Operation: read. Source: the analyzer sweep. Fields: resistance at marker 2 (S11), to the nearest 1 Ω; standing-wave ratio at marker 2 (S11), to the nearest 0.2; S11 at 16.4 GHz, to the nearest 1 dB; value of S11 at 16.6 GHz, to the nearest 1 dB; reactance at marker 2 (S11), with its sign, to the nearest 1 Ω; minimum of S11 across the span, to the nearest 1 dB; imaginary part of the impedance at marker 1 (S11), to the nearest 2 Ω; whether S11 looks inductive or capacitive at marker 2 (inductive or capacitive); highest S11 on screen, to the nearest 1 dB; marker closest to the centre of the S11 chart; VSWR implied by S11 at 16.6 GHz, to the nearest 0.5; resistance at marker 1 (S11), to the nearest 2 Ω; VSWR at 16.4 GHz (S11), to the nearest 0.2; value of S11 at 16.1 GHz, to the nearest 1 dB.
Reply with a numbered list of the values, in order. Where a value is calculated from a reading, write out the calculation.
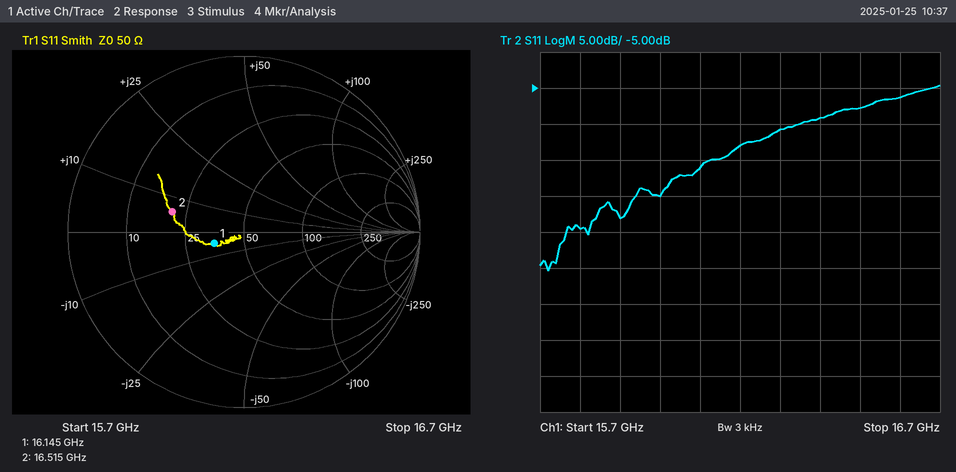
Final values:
1. 21 Ω
2. 2.4
3. -9 dB
4. -6 dB
5. +6 Ω
6. -30 dB
7. -4 Ω
8. inductive
9. -5 dB
10. marker 1
11. |Γ| = 10^(-6/20) = 0.5012; VSWR = (1 + 0.5012)/(1 − 0.5012) ≈ 3.0
12. 36 Ω
13. |Γ| = 10^(-9/20) = 0.3548; VSWR = (1 + 0.3548)/(1 − 0.3548) ≈ 2.10, so 2.0 to the nearest 0.2
14. -16 dB
